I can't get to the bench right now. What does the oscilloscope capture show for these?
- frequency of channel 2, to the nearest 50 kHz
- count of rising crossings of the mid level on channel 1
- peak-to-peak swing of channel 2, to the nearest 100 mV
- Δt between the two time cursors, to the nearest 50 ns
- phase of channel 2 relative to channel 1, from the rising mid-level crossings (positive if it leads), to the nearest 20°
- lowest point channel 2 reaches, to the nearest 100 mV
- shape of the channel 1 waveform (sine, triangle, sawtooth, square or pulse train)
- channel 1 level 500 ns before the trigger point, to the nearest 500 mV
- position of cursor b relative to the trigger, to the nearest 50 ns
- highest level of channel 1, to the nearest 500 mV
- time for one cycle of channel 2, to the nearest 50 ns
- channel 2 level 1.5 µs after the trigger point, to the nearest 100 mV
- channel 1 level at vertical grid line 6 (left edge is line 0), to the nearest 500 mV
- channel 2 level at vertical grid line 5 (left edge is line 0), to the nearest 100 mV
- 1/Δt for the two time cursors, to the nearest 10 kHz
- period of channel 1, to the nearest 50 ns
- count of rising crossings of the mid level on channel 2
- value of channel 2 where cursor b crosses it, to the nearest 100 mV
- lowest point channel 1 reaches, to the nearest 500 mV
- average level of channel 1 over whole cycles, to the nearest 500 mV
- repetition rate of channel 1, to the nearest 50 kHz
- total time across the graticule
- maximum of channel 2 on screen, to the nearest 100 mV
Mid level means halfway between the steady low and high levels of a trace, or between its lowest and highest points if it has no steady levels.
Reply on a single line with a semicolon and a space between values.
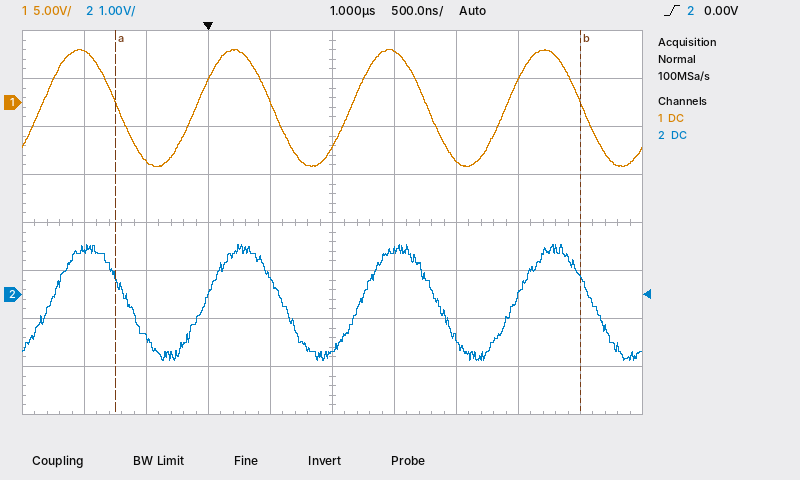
800 kHz; 4; 2.4 V; 3.75 µs; -20°; -1.4 V; sine; -6.0 V; +3.00 µs; 5.5 V; 1.25 µs; 900 mV; 5.5 V; -1.2 V; 270 kHz; 1.25 µs; 4; 400 mV; -6.5 V; -500 mV; 800 kHz; 5 µs; 1.0 V
